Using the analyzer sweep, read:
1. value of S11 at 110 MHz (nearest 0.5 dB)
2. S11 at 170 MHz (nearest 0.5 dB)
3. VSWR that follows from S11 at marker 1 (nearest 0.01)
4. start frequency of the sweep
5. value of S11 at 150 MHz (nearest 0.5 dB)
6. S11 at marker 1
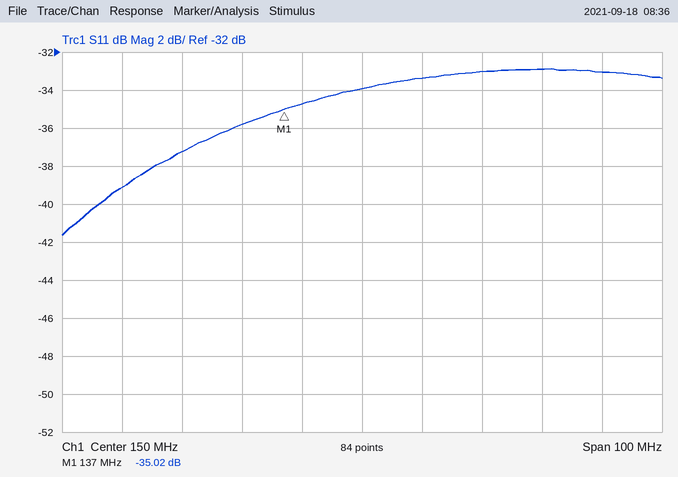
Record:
-39.0 dB
-33.0 dB
1.04
100 MHz
-34.0 dB
-35.02 dB
